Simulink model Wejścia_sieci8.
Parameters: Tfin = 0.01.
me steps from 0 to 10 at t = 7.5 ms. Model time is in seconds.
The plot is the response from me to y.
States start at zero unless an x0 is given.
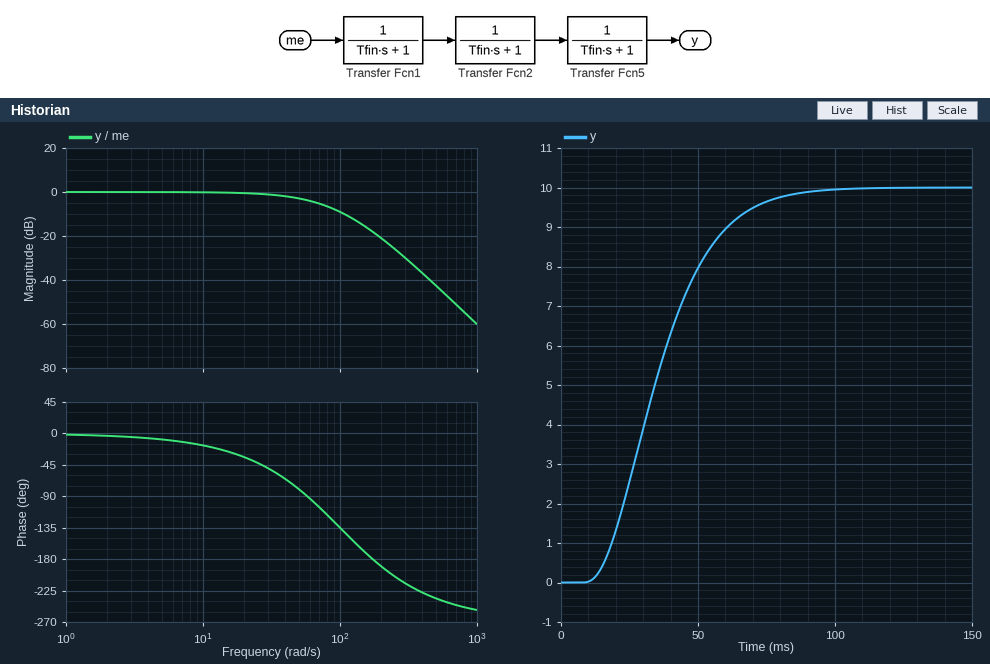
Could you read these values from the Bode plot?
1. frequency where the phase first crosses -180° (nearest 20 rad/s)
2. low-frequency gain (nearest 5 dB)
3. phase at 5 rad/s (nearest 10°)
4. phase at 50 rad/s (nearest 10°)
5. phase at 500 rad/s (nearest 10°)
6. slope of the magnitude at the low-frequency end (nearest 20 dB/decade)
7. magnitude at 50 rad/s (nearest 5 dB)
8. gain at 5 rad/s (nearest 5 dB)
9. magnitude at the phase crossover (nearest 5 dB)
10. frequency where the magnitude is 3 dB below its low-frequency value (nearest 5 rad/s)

180 rad/s
0 dB
-10°
-80°
-240°
0 dB/decade
-5 dB
0 dB
-20 dB
50 rad/s
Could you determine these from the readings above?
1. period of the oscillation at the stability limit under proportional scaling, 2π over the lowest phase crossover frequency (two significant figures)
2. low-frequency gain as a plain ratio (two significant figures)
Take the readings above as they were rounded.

0.035 s
1.0
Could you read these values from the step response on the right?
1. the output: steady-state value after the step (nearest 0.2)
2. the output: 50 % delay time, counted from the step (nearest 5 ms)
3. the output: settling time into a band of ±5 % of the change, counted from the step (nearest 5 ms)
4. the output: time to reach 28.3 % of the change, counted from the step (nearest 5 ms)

10.0
25 ms
65 ms
20 ms
